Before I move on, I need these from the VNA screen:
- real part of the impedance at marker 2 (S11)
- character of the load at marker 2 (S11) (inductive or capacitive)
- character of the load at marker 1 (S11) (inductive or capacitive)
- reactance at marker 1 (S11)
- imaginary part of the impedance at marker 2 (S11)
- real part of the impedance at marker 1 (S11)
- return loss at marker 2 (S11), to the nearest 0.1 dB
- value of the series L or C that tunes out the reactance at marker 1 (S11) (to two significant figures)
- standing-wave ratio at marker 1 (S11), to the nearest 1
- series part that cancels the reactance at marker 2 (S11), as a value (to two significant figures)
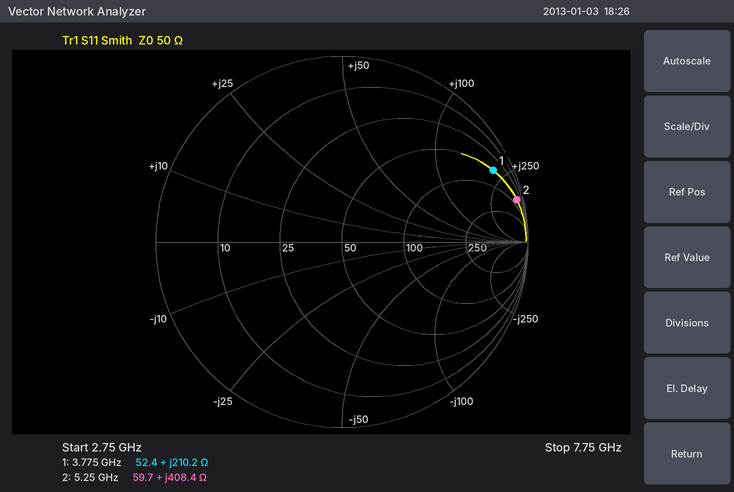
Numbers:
59.7 Ω
inductive
inductive
+210.2 Ω
+408.4 Ω
52.4 Ω
0.3 dB
200 fF
19
74 fF
